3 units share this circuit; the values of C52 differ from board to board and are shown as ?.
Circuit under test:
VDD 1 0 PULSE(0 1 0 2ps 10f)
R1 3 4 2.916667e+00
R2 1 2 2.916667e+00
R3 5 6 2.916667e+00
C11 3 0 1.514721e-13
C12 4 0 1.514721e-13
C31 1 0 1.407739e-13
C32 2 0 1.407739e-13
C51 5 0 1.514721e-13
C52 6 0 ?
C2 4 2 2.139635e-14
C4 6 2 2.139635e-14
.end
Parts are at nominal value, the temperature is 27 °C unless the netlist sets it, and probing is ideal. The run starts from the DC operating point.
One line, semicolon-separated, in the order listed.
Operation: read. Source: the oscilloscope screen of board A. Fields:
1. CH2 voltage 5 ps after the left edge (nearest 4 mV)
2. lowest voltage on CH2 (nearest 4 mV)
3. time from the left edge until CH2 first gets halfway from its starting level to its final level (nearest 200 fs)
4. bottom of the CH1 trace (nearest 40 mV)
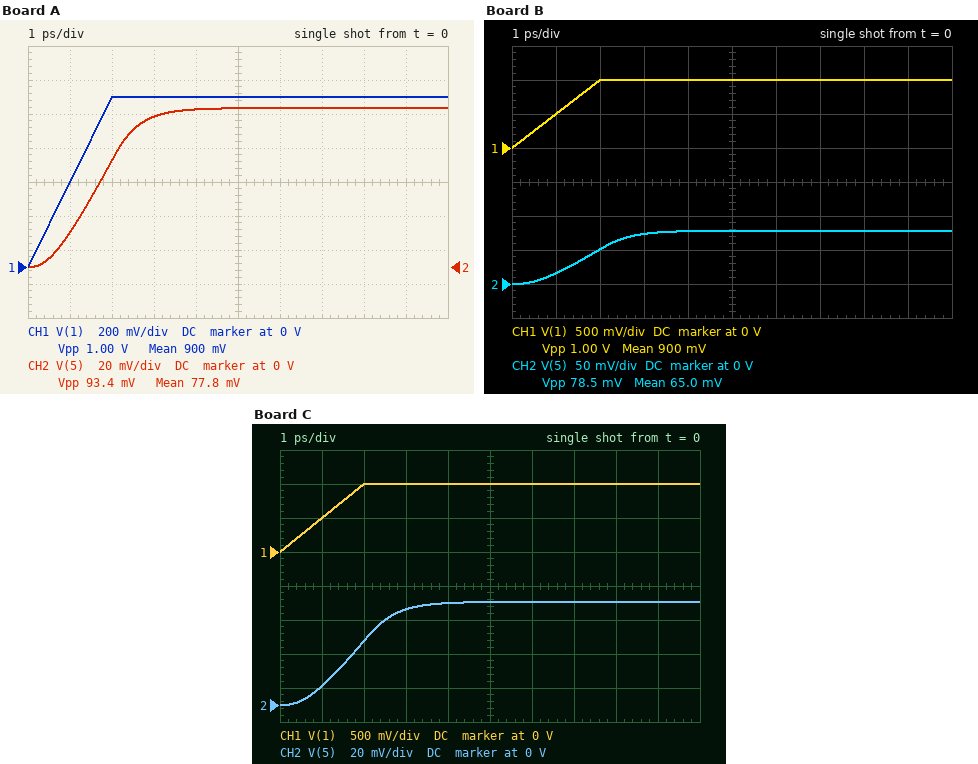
92 mV; 0 V; 1.6 ps; 0 V
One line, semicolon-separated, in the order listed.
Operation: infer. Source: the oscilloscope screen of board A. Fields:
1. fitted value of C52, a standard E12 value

56 fF
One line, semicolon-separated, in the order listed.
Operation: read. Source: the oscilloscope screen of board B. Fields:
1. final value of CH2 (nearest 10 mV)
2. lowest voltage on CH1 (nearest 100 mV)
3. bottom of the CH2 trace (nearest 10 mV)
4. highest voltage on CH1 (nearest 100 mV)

80 mV; 0 V; 0 V; 1.0 V
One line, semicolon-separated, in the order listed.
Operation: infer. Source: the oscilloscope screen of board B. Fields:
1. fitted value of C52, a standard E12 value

100 fF
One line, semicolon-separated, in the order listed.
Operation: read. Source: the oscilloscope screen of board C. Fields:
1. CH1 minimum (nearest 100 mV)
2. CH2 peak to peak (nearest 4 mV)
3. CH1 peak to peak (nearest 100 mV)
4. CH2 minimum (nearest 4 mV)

0 V; 60 mV; 1.0 V; 0 V
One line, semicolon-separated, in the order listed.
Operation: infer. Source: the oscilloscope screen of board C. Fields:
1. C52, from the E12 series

180 fF
